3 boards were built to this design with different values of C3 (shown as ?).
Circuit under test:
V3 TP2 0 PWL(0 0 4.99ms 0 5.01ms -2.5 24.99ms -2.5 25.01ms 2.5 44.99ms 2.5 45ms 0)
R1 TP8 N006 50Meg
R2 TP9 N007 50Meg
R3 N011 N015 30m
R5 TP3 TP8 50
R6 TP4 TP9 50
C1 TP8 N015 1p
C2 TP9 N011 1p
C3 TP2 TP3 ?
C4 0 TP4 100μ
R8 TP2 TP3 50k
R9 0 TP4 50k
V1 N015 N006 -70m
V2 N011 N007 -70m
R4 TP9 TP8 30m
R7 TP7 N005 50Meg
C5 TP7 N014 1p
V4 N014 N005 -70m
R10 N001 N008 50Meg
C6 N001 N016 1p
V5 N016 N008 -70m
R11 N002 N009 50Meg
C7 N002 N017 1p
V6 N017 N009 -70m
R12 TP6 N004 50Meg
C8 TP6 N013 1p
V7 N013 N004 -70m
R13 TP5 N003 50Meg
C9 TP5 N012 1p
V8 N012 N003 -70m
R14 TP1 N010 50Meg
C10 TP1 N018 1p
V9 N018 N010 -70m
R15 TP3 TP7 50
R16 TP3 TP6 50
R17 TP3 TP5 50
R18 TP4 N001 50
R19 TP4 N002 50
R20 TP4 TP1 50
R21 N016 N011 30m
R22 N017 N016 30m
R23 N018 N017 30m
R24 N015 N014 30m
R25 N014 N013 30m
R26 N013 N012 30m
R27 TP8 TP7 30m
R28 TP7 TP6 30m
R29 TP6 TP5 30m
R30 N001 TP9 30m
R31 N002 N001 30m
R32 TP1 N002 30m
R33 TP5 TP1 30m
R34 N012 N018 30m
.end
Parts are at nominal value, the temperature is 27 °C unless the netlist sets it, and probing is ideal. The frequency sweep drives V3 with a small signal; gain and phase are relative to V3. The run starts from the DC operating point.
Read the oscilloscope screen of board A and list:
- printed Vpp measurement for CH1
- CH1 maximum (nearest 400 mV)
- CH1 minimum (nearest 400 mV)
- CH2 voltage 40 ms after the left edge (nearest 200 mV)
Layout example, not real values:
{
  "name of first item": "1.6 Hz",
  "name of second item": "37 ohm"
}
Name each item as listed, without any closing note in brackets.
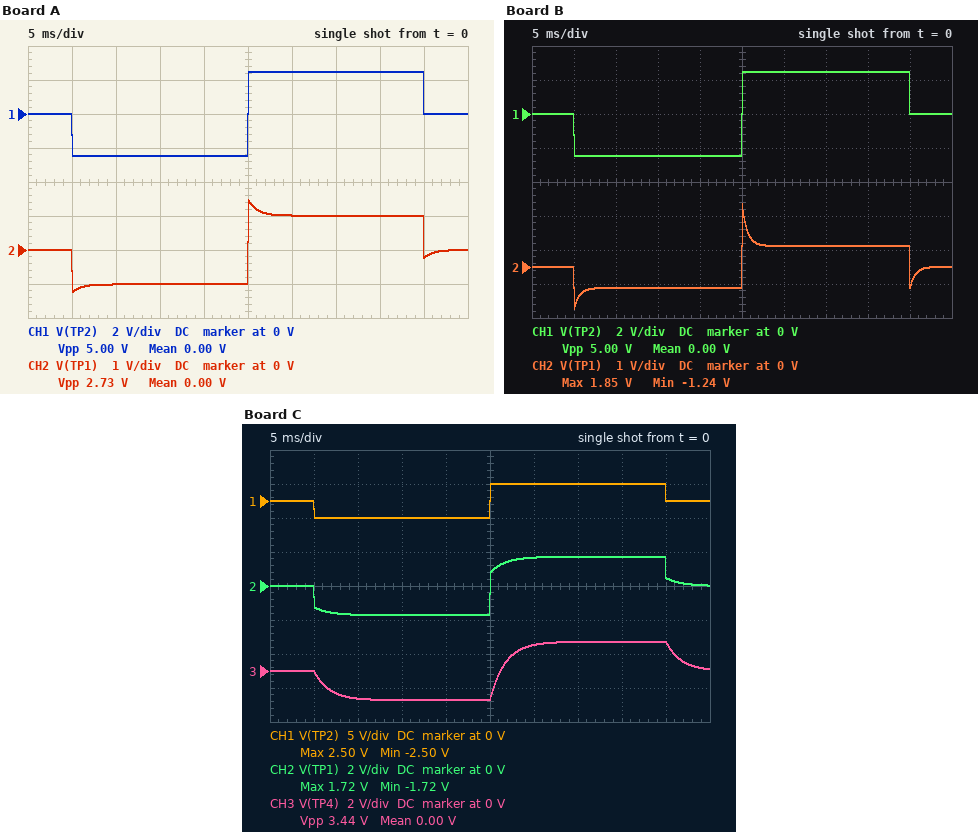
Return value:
{
  "printed Vpp measurement for CH1": "5.00 V",
  "CH1 maximum": "2.4 V",
  "CH1 minimum": "-2.4 V",
  "CH2 voltage 40 ms after the left edge": "1.0 V"
}
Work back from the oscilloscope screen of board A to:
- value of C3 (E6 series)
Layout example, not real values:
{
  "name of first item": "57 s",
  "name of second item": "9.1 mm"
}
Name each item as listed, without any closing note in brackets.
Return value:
{
  "value of C3": "68 µF"
}
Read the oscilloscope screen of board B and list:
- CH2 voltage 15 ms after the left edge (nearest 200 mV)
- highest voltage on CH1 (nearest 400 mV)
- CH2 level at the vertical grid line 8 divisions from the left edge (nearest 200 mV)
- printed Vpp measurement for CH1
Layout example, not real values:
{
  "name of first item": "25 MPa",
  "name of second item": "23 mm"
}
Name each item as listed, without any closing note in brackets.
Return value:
{
  "CH2 voltage 15 ms after the left edge": "-600 mV",
  "highest voltage on CH1": "2.4 V",
  "CH2 level at the vertical grid line 8 divisions from the left edge": "600 mV",
  "printed Vpp measurement for CH1": "5.00 V"
}
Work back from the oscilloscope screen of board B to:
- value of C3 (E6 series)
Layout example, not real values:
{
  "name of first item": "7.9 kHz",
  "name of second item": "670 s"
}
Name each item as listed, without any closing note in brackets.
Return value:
{
  "value of C3": "33 µF"
}
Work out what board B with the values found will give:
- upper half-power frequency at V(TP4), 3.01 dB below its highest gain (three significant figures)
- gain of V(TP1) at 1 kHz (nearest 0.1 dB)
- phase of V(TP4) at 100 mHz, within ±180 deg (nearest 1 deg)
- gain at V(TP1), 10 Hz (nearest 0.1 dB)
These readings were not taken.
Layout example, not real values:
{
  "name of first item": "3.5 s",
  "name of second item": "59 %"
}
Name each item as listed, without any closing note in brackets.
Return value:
{
  "upper half-power frequency at V(TP4), 3.01 dB below its highest gain": "67.2 mHz",
  "gain of V(TP1) at 1 kHz": "-6.2 dB",
  "phase of V(TP4) at 100 mHz, within ±180 deg": "-18 deg",
  "gain at V(TP1), 10 Hz": "-12.1 dB"
}
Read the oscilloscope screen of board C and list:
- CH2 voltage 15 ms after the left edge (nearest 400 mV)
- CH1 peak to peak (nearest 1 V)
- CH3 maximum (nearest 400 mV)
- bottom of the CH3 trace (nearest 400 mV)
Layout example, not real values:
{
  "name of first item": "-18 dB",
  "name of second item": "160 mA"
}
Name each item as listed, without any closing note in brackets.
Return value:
{
  "CH2 voltage 15 ms after the left edge": "-1.6 V",
  "CH1 peak to peak": "5 V",
  "CH3 maximum": "1.6 V",
  "bottom of the CH3 trace": "-1.6 V"
}
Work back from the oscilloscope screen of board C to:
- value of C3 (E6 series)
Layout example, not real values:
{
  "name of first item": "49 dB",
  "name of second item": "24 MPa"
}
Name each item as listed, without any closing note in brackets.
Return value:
{
  "value of C3": "220 µF"
}
